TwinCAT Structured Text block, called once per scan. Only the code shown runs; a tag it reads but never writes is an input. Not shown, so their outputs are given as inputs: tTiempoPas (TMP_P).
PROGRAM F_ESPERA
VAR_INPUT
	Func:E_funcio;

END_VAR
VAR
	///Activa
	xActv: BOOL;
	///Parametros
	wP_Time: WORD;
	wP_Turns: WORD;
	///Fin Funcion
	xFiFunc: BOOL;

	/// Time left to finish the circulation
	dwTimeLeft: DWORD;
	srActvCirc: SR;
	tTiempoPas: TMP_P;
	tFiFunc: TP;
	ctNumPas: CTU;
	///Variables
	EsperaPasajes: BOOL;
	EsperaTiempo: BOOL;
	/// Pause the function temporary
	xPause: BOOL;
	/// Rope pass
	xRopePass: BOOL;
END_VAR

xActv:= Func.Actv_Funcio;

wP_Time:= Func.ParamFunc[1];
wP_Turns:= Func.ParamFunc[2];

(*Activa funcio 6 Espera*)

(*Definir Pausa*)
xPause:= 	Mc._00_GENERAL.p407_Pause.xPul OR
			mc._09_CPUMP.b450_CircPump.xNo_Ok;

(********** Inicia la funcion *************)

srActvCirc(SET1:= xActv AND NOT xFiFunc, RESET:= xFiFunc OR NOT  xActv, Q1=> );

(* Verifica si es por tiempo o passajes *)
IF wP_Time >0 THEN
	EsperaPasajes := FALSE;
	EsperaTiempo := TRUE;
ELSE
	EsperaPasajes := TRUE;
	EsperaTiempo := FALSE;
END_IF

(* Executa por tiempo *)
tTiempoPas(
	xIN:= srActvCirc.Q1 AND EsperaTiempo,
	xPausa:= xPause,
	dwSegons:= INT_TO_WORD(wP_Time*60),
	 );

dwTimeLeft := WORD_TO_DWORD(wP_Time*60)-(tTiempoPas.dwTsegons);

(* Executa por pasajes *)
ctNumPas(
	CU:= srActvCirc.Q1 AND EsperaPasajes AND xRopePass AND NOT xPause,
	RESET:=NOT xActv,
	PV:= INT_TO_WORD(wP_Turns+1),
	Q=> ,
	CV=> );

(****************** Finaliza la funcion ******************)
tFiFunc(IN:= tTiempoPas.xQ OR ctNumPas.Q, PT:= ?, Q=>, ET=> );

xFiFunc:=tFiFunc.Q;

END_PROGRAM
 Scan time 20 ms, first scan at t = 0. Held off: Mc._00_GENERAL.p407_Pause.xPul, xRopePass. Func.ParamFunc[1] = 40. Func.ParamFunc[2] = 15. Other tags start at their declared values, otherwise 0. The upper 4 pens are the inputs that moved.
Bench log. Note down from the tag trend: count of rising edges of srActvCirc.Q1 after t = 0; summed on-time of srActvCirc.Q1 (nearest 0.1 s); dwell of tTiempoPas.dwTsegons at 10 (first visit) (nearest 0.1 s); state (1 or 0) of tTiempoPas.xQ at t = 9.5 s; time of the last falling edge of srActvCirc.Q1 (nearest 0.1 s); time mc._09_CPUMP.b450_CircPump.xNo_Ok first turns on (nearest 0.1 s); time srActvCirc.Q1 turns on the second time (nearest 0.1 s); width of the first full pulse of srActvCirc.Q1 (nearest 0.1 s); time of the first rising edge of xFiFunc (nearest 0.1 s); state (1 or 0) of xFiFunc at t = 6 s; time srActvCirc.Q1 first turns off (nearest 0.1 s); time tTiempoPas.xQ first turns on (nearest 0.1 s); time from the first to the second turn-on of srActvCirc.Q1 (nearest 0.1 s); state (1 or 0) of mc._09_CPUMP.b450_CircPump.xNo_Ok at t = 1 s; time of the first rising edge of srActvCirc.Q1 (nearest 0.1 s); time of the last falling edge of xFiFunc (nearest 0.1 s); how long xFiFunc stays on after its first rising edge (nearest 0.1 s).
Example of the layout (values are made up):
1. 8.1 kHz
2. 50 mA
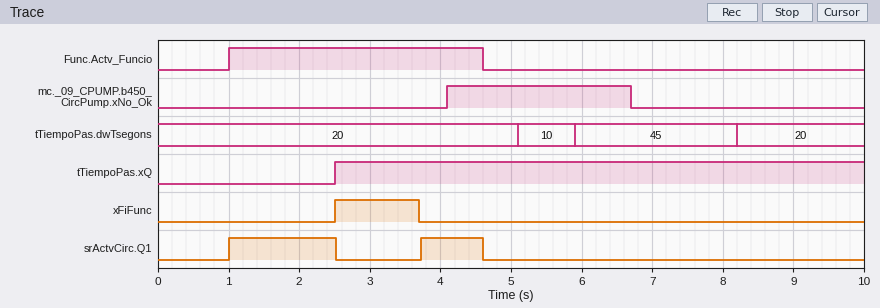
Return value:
1. 2
2. 2.4 s
3. 0.8 s
4. 1
5. 4.6 s
6. 4.1 s
7. 3.7 s
8. 1.5 s
9. 2.5 s
10. 0
11. 2.5 s
12. 2.5 s
13. 2.7 s
14. 0
15. 1.0 s
16. 3.7 s
17. 1.2 s
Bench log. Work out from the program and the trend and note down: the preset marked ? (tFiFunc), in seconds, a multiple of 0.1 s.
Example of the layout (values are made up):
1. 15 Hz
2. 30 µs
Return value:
1. 1.2 s
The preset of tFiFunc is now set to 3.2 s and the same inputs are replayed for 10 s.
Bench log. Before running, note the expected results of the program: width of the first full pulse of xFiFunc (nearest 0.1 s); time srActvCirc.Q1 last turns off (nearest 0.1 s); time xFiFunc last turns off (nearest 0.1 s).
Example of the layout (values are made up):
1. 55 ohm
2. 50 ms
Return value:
1. 3.2 s
2. 2.5 s
3. 5.7 s
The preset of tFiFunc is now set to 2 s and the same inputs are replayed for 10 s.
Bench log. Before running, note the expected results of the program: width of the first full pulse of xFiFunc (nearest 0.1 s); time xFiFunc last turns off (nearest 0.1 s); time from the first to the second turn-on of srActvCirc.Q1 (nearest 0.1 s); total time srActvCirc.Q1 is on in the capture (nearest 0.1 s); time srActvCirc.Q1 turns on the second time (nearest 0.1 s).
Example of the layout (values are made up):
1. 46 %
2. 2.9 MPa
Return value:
1. 2.0 s
2. 4.5 s
3. 3.5 s
4. 1.6 s
5. 4.5 s
